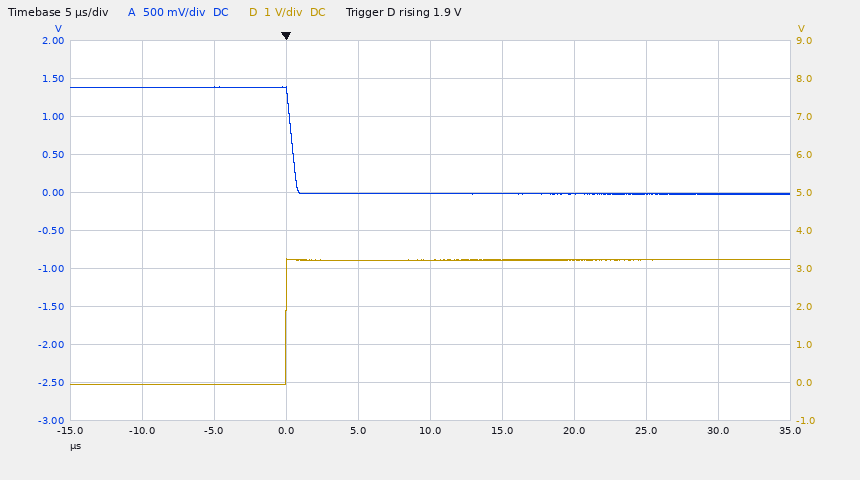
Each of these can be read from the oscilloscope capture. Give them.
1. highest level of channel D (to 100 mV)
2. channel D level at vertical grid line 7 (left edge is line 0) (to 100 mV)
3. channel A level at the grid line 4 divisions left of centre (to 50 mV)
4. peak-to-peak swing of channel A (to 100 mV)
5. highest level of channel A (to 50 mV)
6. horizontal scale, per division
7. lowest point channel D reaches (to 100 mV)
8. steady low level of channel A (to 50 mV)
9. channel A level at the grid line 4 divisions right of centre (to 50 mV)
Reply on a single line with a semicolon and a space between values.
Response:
3.3 V; 3.2 V; 1.40 V; 1.40 V; 1.40 V; 5 µs; -100 mV; 0 mV; 0 mV
